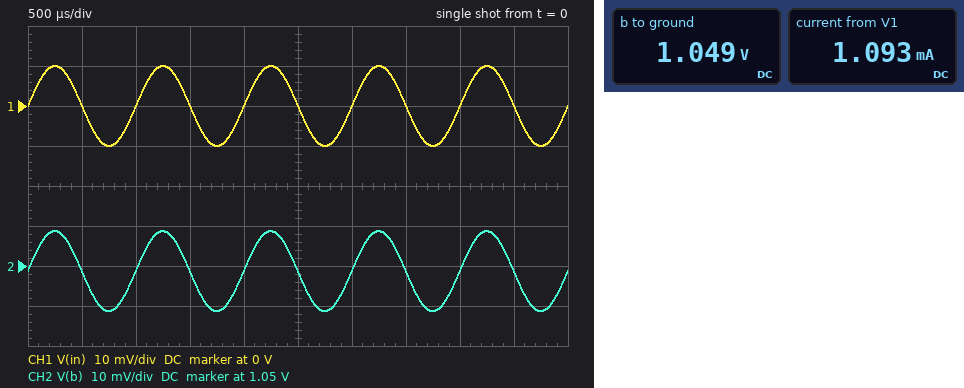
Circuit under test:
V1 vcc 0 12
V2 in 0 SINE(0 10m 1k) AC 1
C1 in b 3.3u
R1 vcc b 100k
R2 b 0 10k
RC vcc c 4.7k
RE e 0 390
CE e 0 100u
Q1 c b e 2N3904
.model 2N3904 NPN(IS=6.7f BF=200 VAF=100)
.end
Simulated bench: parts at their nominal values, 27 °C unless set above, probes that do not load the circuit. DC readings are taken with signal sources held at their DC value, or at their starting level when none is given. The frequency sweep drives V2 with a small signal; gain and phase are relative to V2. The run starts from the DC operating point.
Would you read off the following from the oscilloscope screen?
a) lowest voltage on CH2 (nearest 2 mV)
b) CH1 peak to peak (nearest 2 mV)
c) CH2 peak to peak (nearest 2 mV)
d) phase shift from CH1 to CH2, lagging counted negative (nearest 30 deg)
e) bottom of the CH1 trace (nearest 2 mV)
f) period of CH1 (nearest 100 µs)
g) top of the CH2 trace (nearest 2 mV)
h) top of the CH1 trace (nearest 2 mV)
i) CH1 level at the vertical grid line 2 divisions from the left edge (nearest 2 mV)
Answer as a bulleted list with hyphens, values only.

- 1.038 V
- 20 mV
- 20 mV
- 0 deg
- -10 mV
- 1.0 ms
- 1.058 V
- 10 mV
- 0 V
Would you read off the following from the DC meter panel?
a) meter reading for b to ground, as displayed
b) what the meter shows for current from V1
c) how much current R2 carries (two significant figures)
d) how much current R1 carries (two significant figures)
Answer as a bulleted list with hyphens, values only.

- 1.049 V
- 1.093 mA
- 100 µA
- 110 µA
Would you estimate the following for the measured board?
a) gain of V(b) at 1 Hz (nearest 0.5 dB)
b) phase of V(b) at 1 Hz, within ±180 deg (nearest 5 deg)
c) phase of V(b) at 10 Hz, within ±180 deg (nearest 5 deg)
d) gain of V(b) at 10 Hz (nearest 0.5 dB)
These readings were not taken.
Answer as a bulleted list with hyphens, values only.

- -15.5 dB
- 80 deg
- 30 deg
- -2.0 dB
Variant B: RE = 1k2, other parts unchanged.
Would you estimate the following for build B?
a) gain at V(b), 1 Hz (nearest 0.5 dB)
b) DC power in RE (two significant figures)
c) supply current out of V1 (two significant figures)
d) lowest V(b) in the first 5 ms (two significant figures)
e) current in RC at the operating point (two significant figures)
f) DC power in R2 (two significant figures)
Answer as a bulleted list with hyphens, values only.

- -15.0 dB
- 160 µW
- 470 µA
- 1.1 V
- 360 µA
- 120 µW
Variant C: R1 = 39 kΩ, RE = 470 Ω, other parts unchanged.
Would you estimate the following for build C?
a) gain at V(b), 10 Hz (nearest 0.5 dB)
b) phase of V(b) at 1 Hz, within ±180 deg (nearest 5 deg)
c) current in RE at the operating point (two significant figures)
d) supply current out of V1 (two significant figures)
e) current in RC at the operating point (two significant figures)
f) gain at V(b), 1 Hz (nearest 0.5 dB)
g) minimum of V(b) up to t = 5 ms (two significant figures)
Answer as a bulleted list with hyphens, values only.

- -29.5 dB
- 75 deg
- 2.4 mA
- 2.6 mA
- 2.3 mA
- -41.0 dB
- 1.8 V
